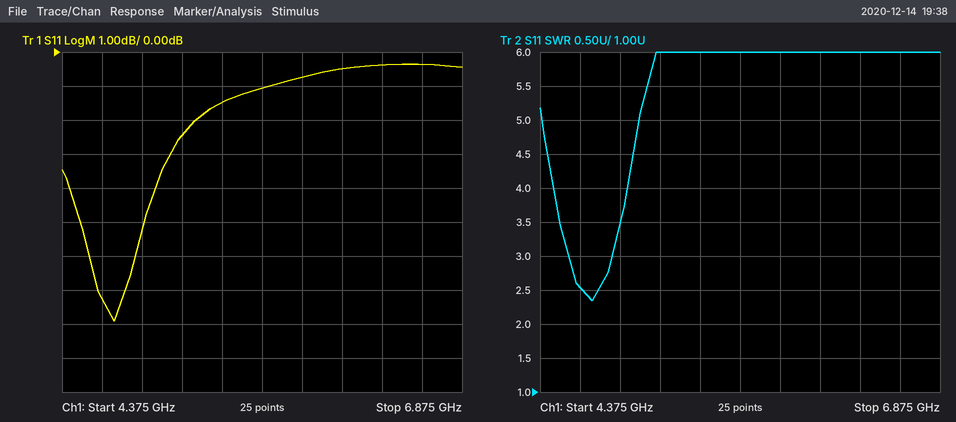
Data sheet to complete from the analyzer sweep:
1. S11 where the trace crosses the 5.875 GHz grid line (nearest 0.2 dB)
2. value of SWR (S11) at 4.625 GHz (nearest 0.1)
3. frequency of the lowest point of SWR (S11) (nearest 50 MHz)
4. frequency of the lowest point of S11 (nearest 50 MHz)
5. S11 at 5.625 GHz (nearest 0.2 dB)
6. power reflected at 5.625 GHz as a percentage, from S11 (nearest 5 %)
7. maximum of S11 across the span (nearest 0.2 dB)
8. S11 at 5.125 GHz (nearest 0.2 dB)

-0.8 dB
2.5
4.70 GHz
4.70 GHz
-1.0 dB
80 %
-0.4 dB
-2.4 dB
